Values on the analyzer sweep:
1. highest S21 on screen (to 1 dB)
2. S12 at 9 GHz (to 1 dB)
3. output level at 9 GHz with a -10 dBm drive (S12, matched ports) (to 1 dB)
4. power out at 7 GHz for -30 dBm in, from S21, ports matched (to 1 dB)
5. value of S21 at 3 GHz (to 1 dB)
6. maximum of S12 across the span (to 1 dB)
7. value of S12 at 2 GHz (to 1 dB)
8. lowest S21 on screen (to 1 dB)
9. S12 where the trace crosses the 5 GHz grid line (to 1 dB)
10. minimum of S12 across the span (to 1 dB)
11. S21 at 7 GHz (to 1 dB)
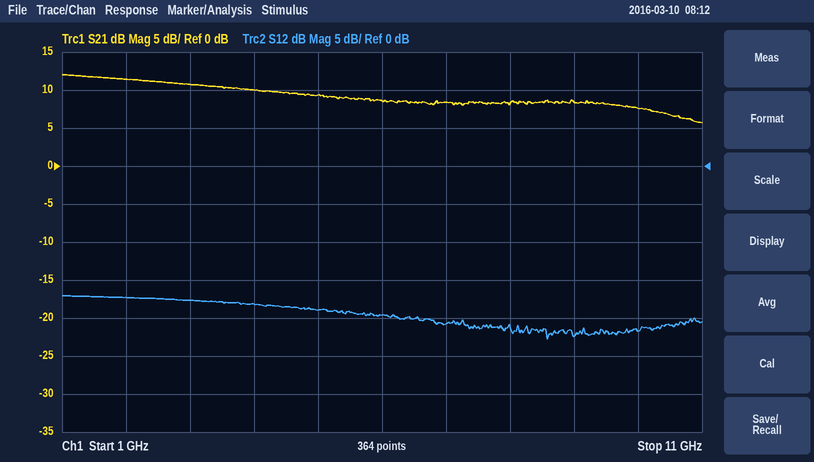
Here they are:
12 dB
-22 dB
-32 dBm
-22 dBm
11 dB
-17 dB
-17 dB
6 dB
-19 dB
-23 dB
8 dB
